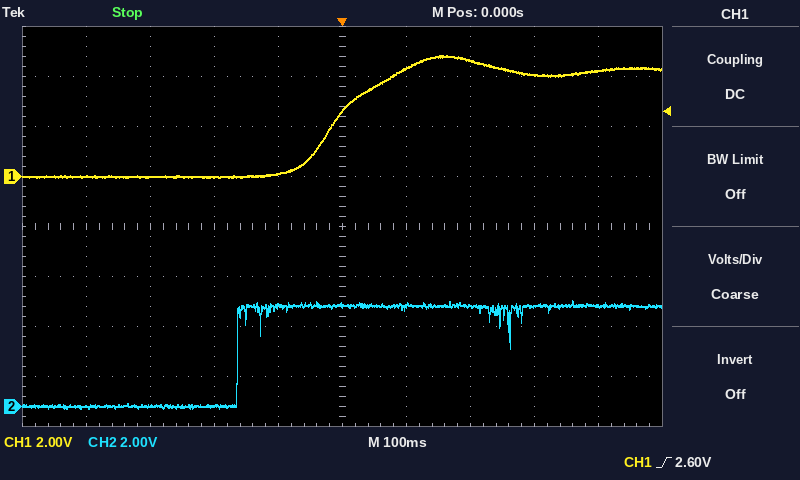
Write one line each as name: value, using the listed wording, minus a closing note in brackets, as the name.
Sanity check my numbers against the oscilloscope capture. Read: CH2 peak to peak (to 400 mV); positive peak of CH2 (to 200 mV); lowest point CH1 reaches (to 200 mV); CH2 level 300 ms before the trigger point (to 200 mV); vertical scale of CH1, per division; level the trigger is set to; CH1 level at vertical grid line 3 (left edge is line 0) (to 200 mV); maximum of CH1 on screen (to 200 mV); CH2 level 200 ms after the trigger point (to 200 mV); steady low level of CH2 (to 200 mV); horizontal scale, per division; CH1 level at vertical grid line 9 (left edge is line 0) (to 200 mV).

CH2 peak to peak: 4.4 V
positive peak of CH2: 4.2 V
lowest point CH1 reaches: 0.0 V
CH2 level 300 ms before the trigger point: 0.0 V
vertical scale of CH1, per division: 2 V
level the trigger is set to: 2.60 V
CH1 level at vertical grid line 3 (left edge is line 0): 0.0 V
maximum of CH1 on screen: 4.8 V
CH2 level 200 ms after the trigger point: 4.0 V
steady low level of CH2: 0.0 V
horizontal scale, per division: 100 ms
CH1 level at vertical grid line 9 (left edge is line 0): 4.2 V
